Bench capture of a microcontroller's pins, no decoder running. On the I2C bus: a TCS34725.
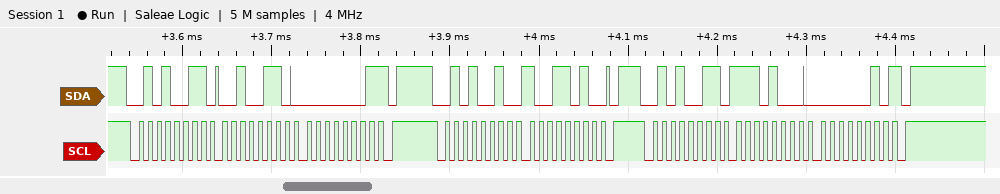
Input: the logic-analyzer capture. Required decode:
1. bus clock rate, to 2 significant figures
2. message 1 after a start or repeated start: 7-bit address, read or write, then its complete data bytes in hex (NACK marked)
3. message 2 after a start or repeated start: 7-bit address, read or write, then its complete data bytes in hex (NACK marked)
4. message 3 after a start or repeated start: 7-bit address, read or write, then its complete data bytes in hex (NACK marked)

100 kHz
0x29 read: 26 01 NACK
0x29 write: 9A
0x29 read: E8 02 NACK
